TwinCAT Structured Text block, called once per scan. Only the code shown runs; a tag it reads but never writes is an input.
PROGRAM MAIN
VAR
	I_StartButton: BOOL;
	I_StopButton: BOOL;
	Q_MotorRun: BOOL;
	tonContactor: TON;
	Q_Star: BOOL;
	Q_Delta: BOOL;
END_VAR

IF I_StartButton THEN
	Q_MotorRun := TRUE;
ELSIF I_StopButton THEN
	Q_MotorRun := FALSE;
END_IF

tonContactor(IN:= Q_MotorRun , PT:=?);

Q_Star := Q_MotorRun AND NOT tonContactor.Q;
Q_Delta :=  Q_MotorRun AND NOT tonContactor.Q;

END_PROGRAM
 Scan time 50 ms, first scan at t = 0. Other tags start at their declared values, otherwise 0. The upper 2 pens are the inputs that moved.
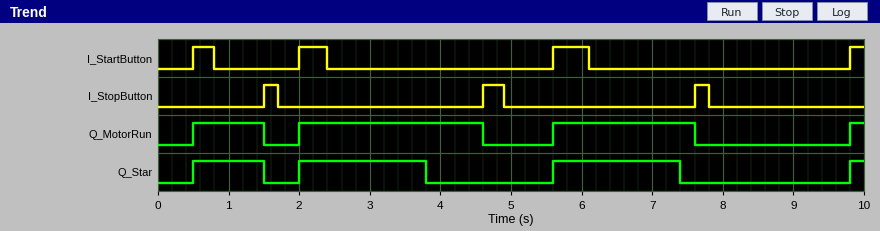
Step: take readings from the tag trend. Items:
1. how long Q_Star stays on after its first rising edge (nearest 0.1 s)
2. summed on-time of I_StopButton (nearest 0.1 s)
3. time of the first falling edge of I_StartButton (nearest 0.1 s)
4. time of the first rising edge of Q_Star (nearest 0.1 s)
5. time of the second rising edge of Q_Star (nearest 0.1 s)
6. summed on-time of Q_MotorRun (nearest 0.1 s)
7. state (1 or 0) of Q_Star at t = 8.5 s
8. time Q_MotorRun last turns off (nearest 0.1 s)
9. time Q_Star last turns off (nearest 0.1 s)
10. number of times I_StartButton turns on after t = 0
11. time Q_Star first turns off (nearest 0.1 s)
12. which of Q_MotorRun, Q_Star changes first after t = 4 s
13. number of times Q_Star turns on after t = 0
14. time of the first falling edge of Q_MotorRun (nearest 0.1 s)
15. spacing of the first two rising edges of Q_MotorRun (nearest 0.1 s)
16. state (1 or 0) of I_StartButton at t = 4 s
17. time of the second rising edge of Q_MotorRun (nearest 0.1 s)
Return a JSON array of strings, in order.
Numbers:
["1.0 s", "0.7 s", "0.8 s", "0.5 s", "2.0 s", "5.8 s", "0", "7.6 s", "7.4 s", "4", "1.5 s", "Q_MotorRun", "4", "1.5 s", "1.5 s", "0", "2.0 s"]
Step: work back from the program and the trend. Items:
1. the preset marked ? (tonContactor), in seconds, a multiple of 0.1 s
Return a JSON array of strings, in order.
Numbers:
["1.8 s"]
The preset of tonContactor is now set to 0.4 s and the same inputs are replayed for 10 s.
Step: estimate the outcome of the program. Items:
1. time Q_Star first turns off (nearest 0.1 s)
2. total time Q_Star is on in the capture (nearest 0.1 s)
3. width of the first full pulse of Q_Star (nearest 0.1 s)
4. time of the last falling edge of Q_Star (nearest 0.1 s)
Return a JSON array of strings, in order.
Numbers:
["0.9 s", "1.4 s", "0.4 s", "6.0 s"]
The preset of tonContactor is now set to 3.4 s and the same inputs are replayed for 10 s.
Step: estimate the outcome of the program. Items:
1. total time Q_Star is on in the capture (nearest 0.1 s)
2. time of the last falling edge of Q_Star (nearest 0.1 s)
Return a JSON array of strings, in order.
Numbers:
["5.8 s", "7.6 s"]
